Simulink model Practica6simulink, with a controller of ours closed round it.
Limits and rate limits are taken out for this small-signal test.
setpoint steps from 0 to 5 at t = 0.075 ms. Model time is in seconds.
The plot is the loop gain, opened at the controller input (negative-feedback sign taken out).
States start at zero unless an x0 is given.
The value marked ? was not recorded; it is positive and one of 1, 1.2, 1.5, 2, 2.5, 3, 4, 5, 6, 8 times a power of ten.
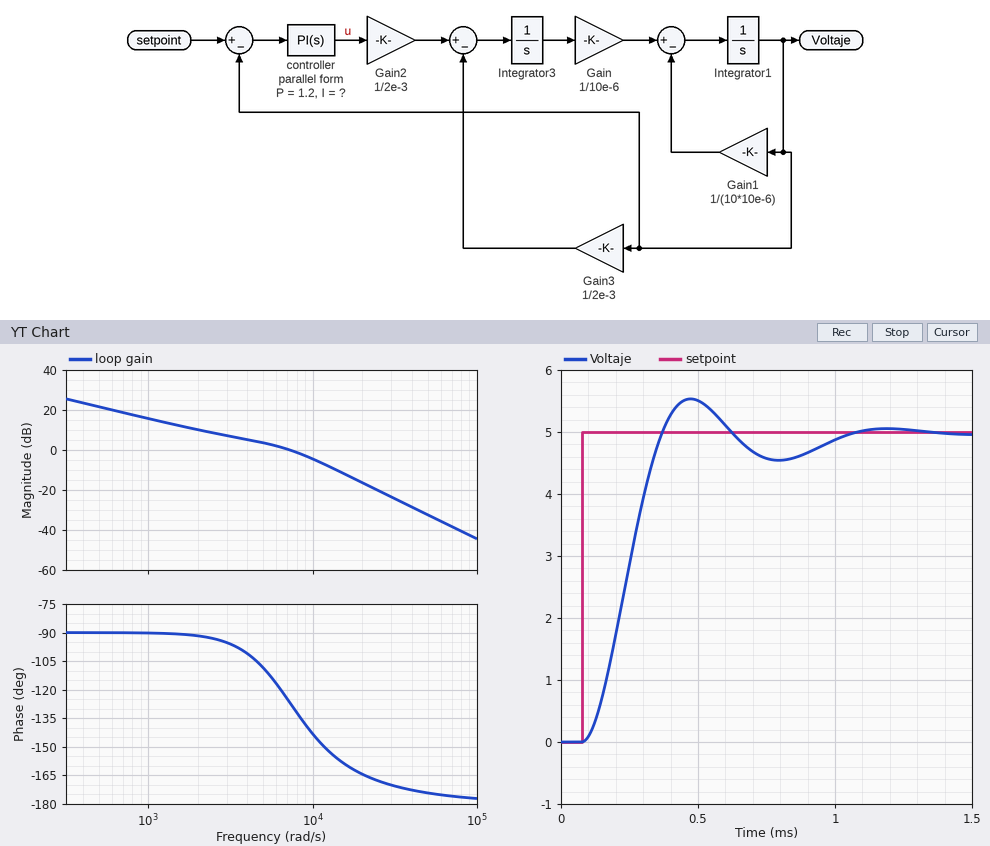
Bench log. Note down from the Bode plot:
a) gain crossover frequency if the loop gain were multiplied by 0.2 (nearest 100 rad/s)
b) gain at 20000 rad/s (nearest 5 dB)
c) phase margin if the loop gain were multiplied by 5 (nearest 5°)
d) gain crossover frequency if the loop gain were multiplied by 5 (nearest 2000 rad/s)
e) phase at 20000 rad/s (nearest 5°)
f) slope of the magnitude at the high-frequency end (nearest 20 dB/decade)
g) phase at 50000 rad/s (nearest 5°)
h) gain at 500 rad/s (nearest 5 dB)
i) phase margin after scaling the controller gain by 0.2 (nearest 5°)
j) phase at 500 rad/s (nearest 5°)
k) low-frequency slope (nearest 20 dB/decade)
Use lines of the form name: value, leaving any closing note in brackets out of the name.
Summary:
gain crossover frequency if the loop gain were multiplied by 0.2: 1200 rad/s
gain at 20000 rad/s: -15 dB
phase margin if the loop gain were multiplied by 5: 20°
gain crossover frequency if the loop gain were multiplied by 5: 18000 rad/s
phase at 20000 rad/s: -165°
slope of the magnitude at the high-frequency end: -40 dB/decade
phase at 50000 rad/s: -175°
gain at 500 rad/s: 20 dB
phase margin after scaling the controller gain by 0.2: 90°
phase at 500 rad/s: -90°
low-frequency slope: -20 dB/decade
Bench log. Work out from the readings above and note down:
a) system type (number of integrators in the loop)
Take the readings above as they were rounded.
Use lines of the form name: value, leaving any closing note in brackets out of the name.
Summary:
system type: 1
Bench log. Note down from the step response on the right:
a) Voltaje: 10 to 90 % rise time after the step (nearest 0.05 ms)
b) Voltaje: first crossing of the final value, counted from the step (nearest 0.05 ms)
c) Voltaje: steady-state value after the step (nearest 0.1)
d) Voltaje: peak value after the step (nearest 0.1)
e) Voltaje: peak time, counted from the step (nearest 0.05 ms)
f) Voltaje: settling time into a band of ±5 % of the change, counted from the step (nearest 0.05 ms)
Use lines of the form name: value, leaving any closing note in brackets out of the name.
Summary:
Voltaje: 10 to 90 % rise time after the step: 0.20 ms
Voltaje: first crossing of the final value, counted from the step: 0.30 ms
Voltaje: steady-state value after the step: 5.0
Voltaje: peak value after the step: 5.5
Voltaje: peak time, counted from the step: 0.40 ms
Voltaje: settling time into a band of ±5 % of the change, counted from the step: 0.85 ms
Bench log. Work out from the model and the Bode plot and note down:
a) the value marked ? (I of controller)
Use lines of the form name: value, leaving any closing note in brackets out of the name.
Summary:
the value marked ?: 6000
